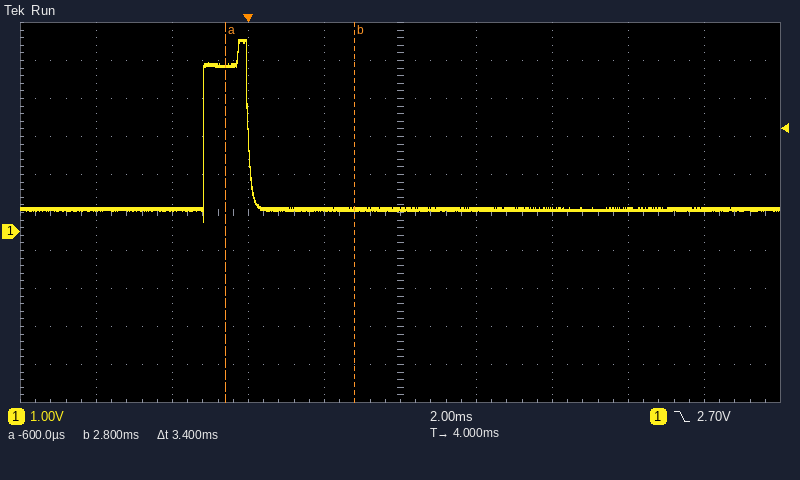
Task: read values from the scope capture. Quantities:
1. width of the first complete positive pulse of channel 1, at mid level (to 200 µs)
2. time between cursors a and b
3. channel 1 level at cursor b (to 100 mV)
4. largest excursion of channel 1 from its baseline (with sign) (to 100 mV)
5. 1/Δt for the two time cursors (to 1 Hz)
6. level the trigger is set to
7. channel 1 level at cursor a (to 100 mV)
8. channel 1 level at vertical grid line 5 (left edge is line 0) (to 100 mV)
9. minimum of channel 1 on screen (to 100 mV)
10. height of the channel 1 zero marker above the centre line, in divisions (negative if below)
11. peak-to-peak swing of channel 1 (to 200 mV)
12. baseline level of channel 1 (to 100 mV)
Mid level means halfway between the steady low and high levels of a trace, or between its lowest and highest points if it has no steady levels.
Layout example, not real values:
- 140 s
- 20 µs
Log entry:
- 1.2 ms
- 3.4 ms
- 600 mV
- +4.5 V
- 294 Hz
- 2.70 V
- 4.4 V
- 600 mV
- 300 mV
- -0.5 div
- 4.8 V
- 600 mV
